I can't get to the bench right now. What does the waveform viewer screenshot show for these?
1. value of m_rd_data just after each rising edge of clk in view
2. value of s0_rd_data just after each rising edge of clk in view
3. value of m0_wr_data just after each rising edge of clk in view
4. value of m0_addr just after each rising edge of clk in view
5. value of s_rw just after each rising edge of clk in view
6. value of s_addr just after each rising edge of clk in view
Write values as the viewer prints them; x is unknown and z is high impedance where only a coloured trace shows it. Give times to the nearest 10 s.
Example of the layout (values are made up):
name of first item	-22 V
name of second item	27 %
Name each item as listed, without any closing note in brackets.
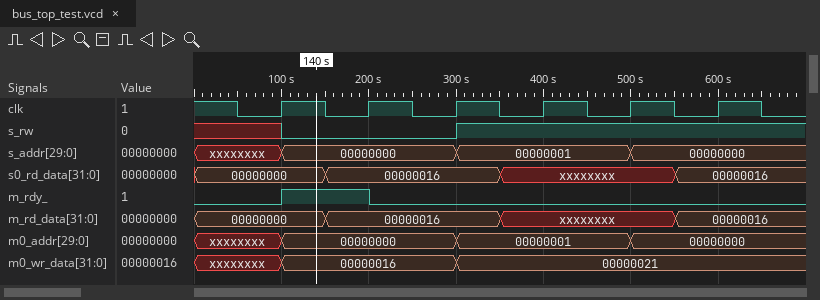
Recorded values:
value of m_rd_data just after each rising edge of clk in view	00000000, 00000016, 00000016, xxxxxxxx, xxxxxxxx, 00000016
value of s0_rd_data just after each rising edge of clk in view	00000000, 00000016, 00000016, xxxxxxxx, xxxxxxxx, 00000016
value of m0_wr_data just after each rising edge of clk in view	00000016, 00000016, 00000021, 00000021, 00000021, 00000021
value of m0_addr just after each rising edge of clk in view	00000000, 00000000, 00000001, 00000001, 00000000, 00000000
value of s_rw just after each rising edge of clk in view	0 0 1 1 1 1
value of s_addr just after each rising edge of clk in view	00000000, 00000000, 00000001, 00000001, 00000000, 00000000
